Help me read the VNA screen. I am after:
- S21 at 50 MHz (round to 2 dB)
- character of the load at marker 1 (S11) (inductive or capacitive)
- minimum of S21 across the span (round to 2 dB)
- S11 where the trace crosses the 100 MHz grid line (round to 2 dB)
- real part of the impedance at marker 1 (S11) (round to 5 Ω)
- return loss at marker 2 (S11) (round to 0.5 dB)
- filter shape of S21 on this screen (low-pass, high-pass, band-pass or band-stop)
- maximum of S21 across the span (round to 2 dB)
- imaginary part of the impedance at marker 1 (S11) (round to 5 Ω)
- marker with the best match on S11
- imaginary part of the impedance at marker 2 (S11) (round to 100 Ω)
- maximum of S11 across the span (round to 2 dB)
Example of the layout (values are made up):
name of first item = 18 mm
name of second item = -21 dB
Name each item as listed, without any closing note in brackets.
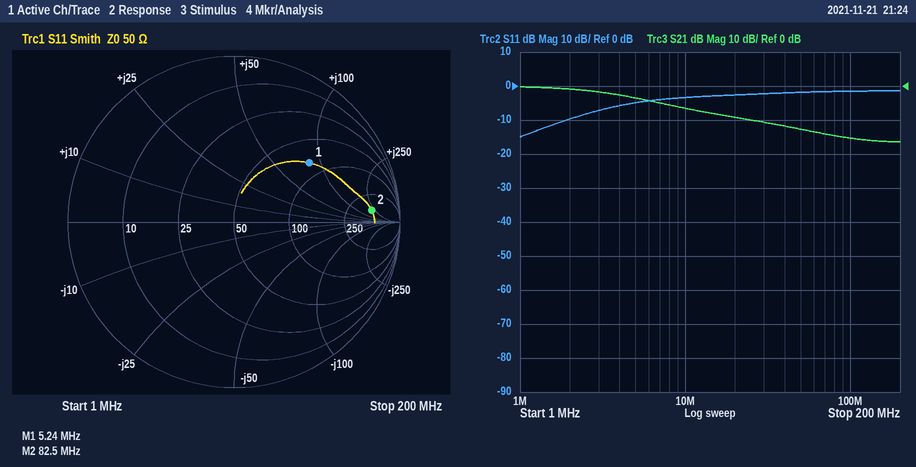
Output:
S21 at 50 MHz = -12 dB
character of the load at marker 1 (S11) = inductive
minimum of S21 across the span = -16 dB
S11 where the trace crosses the 100 MHz grid line = -2 dB
real part of the impedance at marker 1 (S11) = 80 Ω
return loss at marker 2 (S11) = 1.5 dB
filter shape of S21 on this screen = low-pass
maximum of S21 across the span = 0 dB
imaginary part of the impedance at marker 1 (S11) = +85 Ω
marker with the best match on S11 = marker 1
imaginary part of the impedance at marker 2 (S11) = +200 Ω
maximum of S11 across the span = -2 dB
